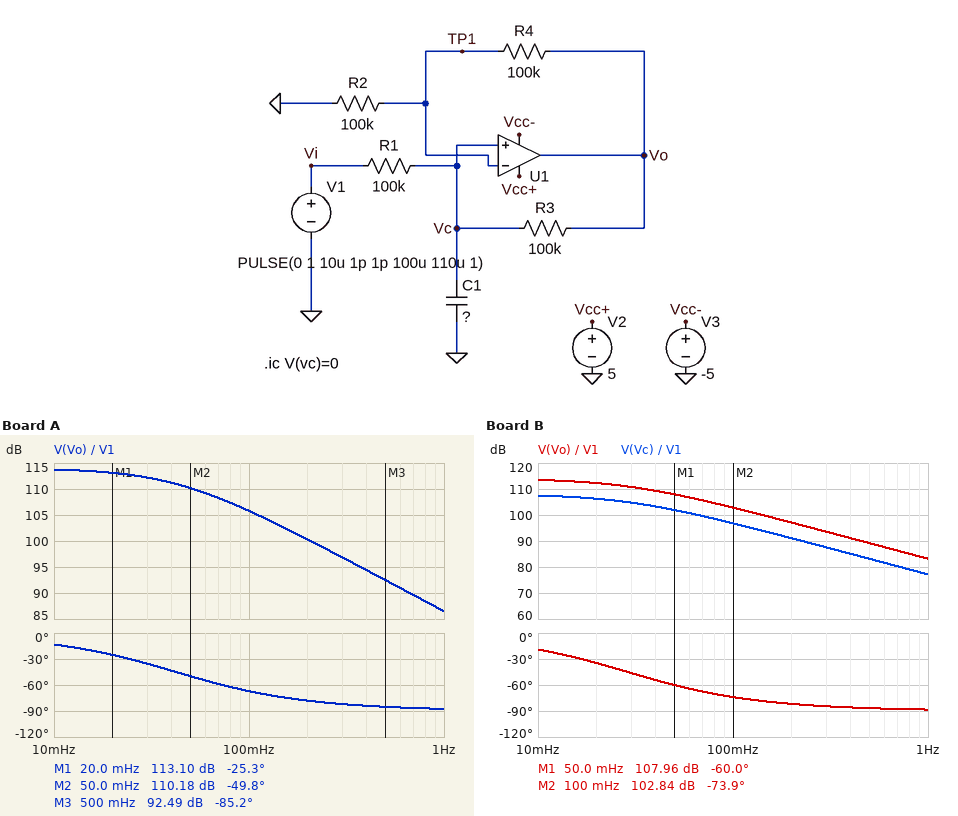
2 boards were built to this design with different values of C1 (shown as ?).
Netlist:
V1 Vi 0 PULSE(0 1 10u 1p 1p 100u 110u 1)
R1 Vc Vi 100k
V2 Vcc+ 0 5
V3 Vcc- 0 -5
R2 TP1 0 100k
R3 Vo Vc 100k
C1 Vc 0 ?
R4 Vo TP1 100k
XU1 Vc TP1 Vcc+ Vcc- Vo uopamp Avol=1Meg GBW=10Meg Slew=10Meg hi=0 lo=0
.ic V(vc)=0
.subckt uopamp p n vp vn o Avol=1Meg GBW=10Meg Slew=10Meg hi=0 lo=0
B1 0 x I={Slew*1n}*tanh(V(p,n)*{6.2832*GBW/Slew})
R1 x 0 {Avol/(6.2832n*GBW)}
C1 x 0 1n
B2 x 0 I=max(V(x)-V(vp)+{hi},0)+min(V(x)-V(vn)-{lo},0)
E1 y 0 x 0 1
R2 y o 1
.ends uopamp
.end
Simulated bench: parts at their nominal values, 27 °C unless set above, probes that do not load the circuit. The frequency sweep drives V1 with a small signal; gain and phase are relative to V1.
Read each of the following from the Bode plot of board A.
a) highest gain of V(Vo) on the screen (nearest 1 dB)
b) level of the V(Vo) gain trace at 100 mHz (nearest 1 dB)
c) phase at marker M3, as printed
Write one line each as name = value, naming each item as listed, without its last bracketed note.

highest gain of V(Vo) on the screen = 114 dB
level of the V(Vo) gain trace at 100 mHz = 106 dB
phase at marker M3, as printed = -85.2 deg
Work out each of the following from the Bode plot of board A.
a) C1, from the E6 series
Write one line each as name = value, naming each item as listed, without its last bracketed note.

C1, from the E6 series = 150 pF
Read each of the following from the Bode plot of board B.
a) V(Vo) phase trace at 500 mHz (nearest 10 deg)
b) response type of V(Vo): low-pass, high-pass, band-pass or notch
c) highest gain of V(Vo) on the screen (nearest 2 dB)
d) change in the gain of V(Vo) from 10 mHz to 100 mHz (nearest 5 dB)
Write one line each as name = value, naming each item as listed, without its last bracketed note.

V(Vo) phase trace at 500 mHz = -90 deg
response type of V(Vo): low-pass, high-pass, band-pass or notch = low-pass
highest gain of V(Vo) on the screen = 114 dB
change in the gain of V(Vo) from 10 mHz to 100 mHz = -10 dB
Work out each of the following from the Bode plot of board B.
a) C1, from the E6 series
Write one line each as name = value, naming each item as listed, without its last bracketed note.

C1, from the E6 series = 220 pF
